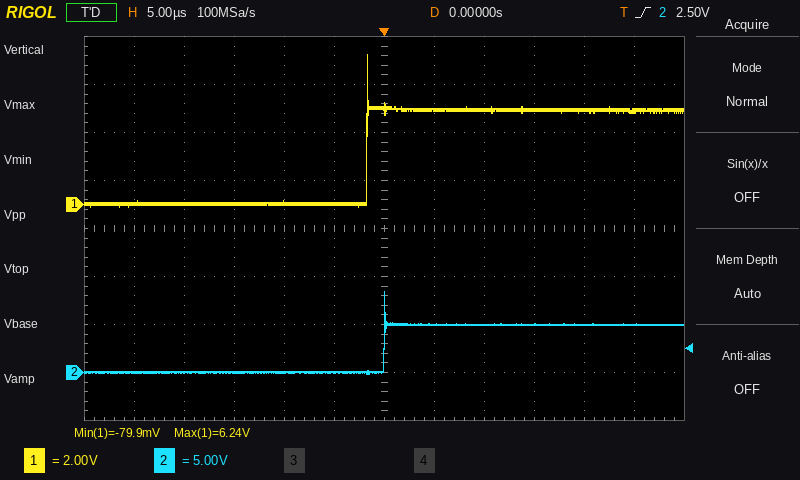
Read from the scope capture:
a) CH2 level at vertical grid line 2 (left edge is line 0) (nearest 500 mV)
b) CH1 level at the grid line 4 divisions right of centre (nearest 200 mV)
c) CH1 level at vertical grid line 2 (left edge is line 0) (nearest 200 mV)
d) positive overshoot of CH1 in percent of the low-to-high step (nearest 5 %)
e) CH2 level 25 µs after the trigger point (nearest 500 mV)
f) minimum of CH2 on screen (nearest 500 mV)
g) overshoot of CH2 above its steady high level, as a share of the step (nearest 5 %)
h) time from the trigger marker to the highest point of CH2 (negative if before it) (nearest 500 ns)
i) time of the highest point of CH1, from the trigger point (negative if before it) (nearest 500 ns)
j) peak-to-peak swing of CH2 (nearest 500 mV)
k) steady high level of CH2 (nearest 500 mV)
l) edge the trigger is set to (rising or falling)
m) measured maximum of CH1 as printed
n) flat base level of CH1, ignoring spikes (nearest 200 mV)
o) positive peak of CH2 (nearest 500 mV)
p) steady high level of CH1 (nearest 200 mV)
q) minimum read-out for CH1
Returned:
0.0 V
4.0 V
0.0 V
60 %
5.0 V
0.0 V
70 %
0.0 µs
-1.5 µs
8.5 V
5.0 V
rising
6.24 V
0.0 V
8.5 V
4.0 V
-79.9 mV
